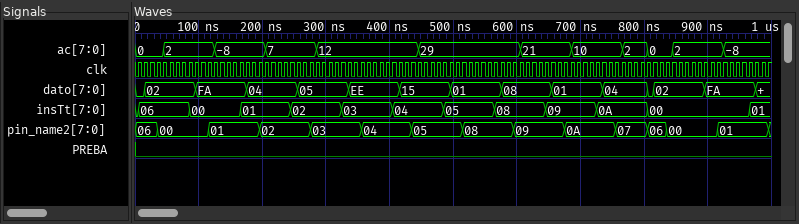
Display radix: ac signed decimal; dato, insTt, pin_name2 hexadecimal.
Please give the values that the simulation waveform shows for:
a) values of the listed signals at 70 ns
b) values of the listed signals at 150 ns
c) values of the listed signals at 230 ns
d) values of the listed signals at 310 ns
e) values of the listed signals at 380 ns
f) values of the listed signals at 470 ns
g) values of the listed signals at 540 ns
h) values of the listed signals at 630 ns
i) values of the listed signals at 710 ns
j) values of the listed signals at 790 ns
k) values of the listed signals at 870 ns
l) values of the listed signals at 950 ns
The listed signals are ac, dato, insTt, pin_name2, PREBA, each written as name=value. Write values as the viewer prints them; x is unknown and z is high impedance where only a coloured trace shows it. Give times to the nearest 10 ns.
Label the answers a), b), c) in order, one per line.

a) ac=2, dato=02, insTt=06, pin_name2=00, PREBA=0
b) ac=-8, dato=FA, insTt=00, pin_name2=01, PREBA=0
c) ac=7, dato=04, insTt=01, pin_name2=02, PREBA=0
d) ac=12, dato=05, insTt=02, pin_name2=03, PREBA=0
e) ac=12, dato=EE, insTt=03, pin_name2=04, PREBA=0
f) ac=29, dato=15, insTt=04, pin_name2=05, PREBA=0
g) ac=29, dato=01, insTt=05, pin_name2=08, PREBA=0
h) ac=21, dato=08, insTt=08, pin_name2=09, PREBA=0
i) ac=10, dato=01, insTt=09, pin_name2=0A, PREBA=0
j) ac=2, dato=04, insTt=0A, pin_name2=07, PREBA=0
k) ac=2, dato=02, insTt=00, pin_name2=00, PREBA=0
l) ac=-8, dato=FA, insTt=00, pin_name2=01, PREBA=0
